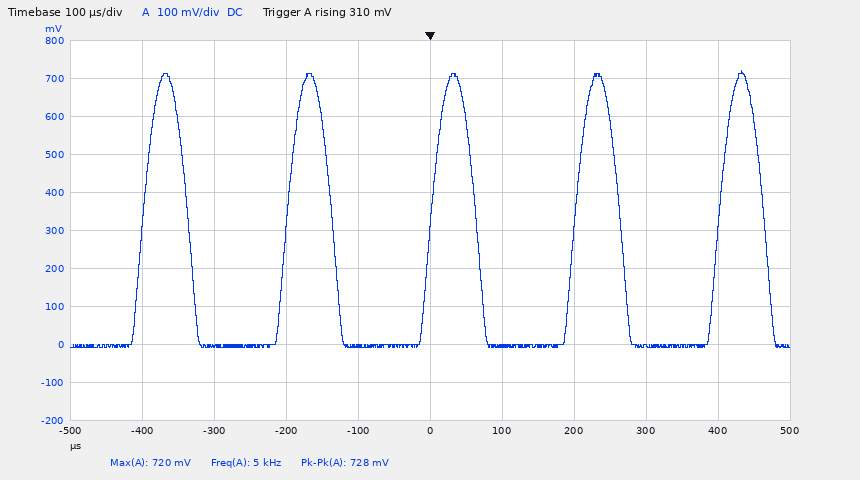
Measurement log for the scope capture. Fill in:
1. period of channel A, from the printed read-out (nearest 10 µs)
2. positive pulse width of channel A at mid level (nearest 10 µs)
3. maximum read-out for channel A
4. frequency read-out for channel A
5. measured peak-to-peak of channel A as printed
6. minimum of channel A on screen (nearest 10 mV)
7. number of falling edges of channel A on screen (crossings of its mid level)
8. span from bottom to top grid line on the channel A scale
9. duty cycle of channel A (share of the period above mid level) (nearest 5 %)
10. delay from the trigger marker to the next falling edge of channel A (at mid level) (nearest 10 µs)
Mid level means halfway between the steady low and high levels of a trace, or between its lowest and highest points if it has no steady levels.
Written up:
200 µs
60 µs
720 mV
5 kHz
728 mV
-10 mV
5
1 V
30 %
60 µs
